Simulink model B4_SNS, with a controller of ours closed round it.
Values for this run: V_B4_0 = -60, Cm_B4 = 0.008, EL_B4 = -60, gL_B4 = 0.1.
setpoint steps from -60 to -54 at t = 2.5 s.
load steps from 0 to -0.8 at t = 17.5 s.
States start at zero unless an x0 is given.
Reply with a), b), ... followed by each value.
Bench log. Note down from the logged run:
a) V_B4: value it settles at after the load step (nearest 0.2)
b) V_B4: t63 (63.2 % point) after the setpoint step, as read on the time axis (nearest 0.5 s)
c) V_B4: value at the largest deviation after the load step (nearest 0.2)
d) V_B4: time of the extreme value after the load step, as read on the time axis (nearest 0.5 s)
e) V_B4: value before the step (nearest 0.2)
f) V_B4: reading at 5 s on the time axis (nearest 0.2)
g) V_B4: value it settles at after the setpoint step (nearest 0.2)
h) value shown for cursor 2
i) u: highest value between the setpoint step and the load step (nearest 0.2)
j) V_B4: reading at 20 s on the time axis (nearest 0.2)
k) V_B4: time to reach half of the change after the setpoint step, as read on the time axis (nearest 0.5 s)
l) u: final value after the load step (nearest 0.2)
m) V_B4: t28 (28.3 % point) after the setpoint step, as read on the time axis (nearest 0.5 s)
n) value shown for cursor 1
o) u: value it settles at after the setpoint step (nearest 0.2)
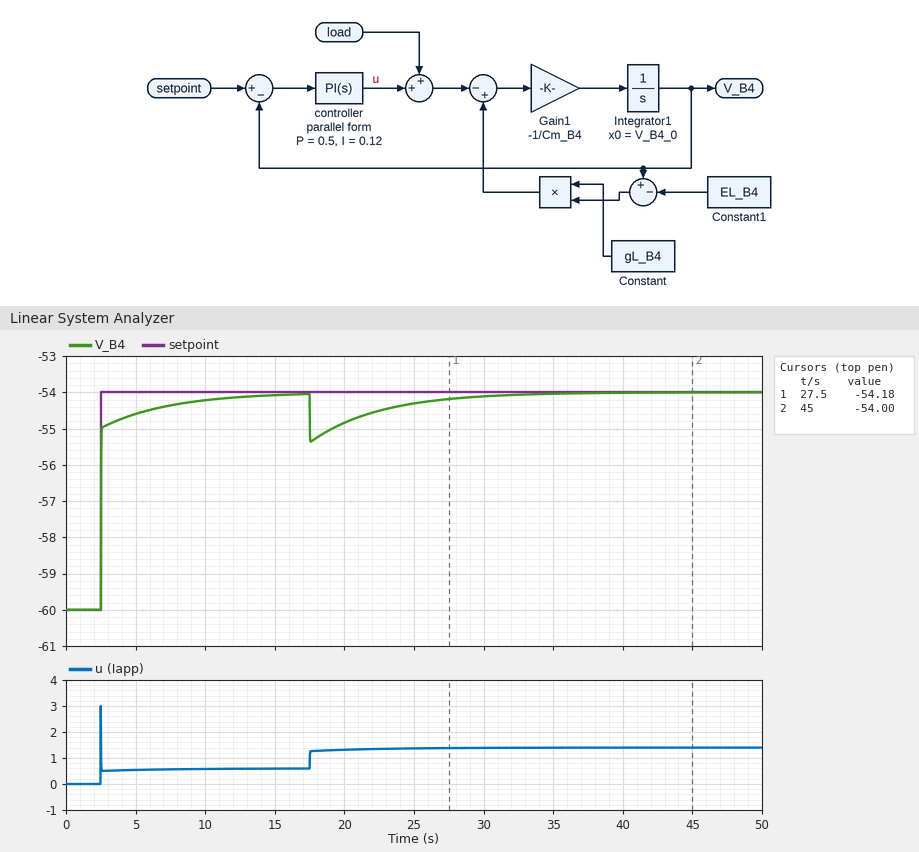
a) -54.0
b) 2.5 s
c) -55.4
d) 17.5 s
e) -60.0
f) -54.6
g) -54.0
h) -54.00
i) 3.0
j) -54.8
k) 2.5 s
l) 1.4
m) 2.5 s
n) -54.18
o) 0.6
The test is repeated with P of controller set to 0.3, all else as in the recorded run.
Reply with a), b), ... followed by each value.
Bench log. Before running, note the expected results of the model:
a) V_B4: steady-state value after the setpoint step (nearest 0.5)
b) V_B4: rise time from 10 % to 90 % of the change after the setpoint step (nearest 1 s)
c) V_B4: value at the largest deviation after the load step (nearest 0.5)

a) -54.0
b) 3 s
c) -56.0
